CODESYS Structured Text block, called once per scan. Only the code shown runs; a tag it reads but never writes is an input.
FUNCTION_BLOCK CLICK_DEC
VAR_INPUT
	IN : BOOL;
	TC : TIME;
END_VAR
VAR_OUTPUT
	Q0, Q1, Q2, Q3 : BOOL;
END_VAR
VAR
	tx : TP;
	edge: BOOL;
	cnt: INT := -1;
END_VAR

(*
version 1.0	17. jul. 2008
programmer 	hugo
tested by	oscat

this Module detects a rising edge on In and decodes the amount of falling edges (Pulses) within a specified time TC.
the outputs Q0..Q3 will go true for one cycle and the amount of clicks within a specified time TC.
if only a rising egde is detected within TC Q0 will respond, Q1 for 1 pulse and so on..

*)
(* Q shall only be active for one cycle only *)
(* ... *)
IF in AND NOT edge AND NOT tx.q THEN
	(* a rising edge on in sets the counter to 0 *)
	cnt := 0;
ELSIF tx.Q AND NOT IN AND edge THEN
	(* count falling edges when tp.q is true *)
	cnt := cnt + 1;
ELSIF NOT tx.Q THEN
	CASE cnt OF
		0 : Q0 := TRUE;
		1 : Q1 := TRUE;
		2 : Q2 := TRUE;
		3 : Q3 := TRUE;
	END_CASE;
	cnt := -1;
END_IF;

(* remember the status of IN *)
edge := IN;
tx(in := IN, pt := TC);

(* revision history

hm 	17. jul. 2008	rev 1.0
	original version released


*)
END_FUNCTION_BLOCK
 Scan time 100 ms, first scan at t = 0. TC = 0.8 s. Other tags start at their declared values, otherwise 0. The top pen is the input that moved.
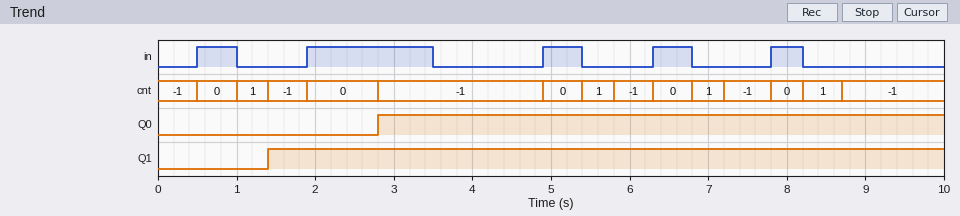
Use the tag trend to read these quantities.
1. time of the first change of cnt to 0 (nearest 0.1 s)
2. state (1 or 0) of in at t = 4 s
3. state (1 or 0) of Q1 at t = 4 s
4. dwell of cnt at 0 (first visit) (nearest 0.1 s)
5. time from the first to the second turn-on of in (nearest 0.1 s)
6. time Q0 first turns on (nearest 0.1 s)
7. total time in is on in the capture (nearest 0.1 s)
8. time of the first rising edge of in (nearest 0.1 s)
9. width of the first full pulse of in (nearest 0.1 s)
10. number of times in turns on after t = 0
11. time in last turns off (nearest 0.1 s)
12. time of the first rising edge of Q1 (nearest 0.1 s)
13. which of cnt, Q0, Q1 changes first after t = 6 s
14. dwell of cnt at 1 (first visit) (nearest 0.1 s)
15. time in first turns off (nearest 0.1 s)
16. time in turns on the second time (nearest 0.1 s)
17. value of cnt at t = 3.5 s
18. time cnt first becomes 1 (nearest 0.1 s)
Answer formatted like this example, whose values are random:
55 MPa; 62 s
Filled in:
0.5 s; 0; 1; 0.5 s; 1.4 s; 2.8 s; 3.5 s; 0.5 s; 0.5 s; 5; 8.2 s; 1.4 s; cnt; 0.4 s; 1.0 s; 1.9 s; -1; 1.0 s
